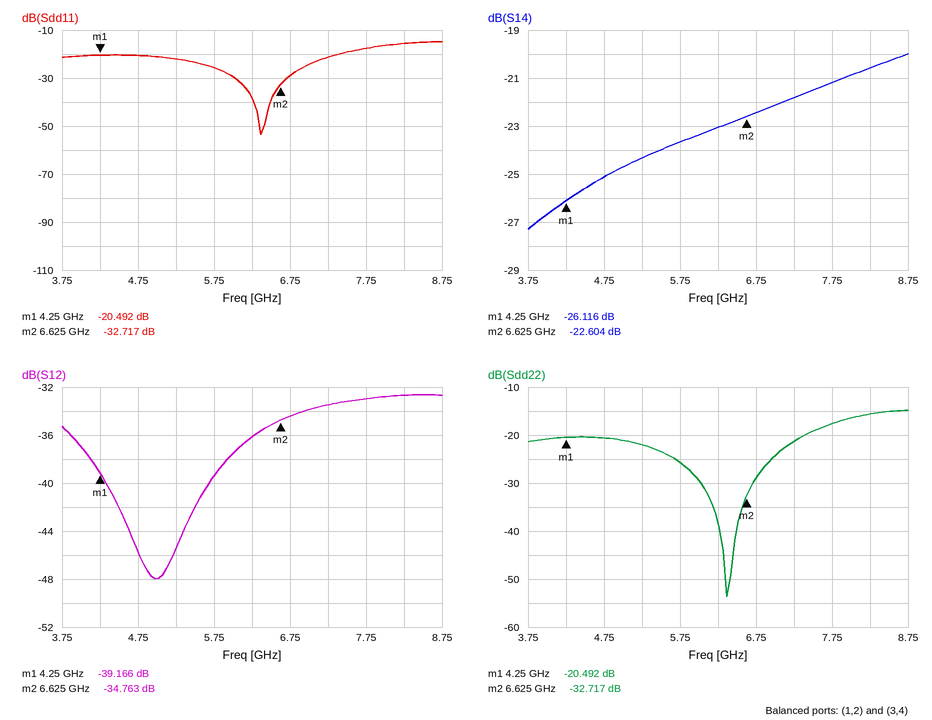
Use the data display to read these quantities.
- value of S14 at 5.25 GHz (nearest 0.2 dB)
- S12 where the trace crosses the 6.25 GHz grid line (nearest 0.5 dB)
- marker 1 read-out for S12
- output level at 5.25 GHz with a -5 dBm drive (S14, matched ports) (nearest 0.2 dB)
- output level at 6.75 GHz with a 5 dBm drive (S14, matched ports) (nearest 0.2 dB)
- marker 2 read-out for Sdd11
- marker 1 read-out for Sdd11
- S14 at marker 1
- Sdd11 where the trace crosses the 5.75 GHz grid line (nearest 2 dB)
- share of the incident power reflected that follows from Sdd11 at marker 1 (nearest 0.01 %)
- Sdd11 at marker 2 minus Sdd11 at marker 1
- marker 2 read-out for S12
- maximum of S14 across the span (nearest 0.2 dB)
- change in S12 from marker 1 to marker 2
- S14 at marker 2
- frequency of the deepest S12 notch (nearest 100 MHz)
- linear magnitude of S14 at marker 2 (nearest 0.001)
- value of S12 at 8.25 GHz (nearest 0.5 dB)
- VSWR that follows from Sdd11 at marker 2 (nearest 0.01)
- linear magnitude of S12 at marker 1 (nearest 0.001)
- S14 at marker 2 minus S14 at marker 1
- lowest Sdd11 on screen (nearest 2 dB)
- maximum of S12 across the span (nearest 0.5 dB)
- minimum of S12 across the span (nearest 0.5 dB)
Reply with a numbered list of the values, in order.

1. -24.4 dB
2. -36.0 dB
3. -39.166 dB
4. -29.4 dBm
5. -17.4 dBm
6. -32.717 dB
7. -20.492 dB
8. -26.116 dB
9. -26 dB
10. 0.89 %
11. -12.225 dB
12. -34.763 dB
13. -20.0 dB
14. 4.403 dB
15. -22.604 dB
16. 5.0 GHz
17. 0.074
18. -32.5 dB
19. 1.05
20. 0.011
21. 3.512 dB
22. -54 dB
23. -32.5 dB
24. -48.0 dB
